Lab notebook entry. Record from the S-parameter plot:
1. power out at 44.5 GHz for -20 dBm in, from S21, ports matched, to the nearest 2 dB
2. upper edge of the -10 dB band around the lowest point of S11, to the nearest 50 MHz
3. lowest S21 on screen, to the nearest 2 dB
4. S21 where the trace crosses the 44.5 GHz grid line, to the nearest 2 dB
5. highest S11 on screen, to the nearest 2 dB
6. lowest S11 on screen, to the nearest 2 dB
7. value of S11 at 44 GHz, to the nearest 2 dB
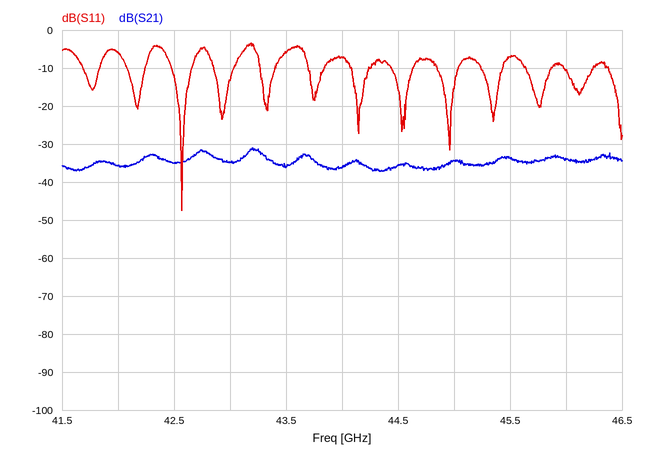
-56 dBm
42.65 GHz
-38 dB
-36 dB
-4 dB
-48 dB
-8 dB
